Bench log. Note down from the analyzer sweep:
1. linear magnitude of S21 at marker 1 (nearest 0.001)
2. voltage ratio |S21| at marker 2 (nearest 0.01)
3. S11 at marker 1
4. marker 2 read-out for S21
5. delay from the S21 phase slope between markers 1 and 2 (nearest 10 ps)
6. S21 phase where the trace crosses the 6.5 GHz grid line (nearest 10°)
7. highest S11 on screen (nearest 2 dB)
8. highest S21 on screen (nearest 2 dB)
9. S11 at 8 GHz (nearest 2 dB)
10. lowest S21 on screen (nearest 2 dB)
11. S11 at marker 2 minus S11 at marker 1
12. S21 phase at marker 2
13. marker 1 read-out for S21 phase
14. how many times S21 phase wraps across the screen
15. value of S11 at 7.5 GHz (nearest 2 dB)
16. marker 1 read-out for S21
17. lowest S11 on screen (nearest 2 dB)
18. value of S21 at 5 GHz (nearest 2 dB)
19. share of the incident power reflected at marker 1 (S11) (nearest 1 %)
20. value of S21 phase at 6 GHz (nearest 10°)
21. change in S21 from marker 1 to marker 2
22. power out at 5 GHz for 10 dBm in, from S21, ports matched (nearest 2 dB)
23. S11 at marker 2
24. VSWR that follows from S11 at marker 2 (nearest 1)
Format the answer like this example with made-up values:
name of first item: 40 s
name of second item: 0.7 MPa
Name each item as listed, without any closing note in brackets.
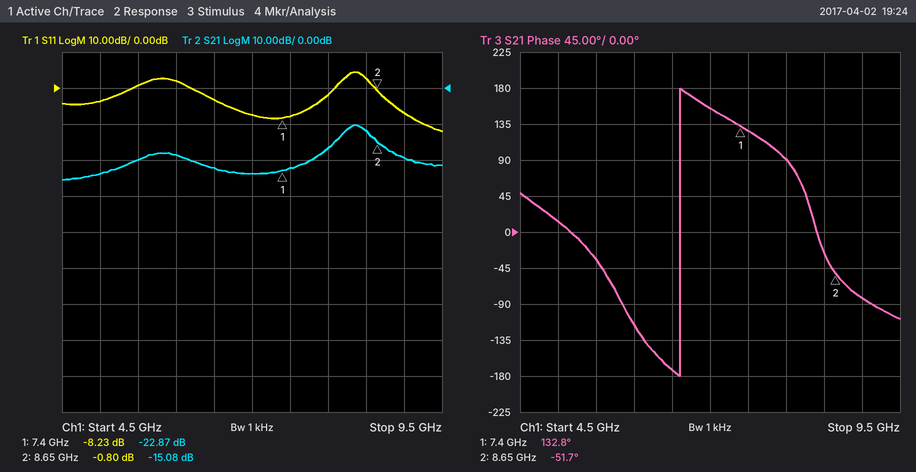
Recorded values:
linear magnitude of S21 at marker 1: 0.072
voltage ratio |S21| at marker 2: 0.18
S11 at marker 1: -8.23 dB
marker 2 read-out for S21: -15.08 dB
delay from the S21 phase slope between markers 1 and 2: 410 ps
S21 phase where the trace crosses the 6.5 GHz grid line: -170°
highest S11 on screen: 4 dB
highest S21 on screen: -10 dB
S11 at 8 GHz: -2 dB
lowest S21 on screen: -26 dB
S11 at marker 2 minus S11 at marker 1: 7.43 dB
S21 phase at marker 2: -51.7°
marker 1 read-out for S21 phase: 132.8°
how many times S21 phase wraps across the screen: 1
value of S11 at 7.5 GHz: -8 dB
marker 1 read-out for S21: -22.87 dB
lowest S11 on screen: -12 dB
value of S21 at 5 GHz: -24 dB
share of the incident power reflected at marker 1 (S11): 15 %
value of S21 phase at 6 GHz: -120°
change in S21 from marker 1 to marker 2: 7.79 dB
power out at 5 GHz for 10 dBm in, from S21, ports matched: -14 dBm
S11 at marker 2: -0.80 dB
VSWR that follows from S11 at marker 2: 22
